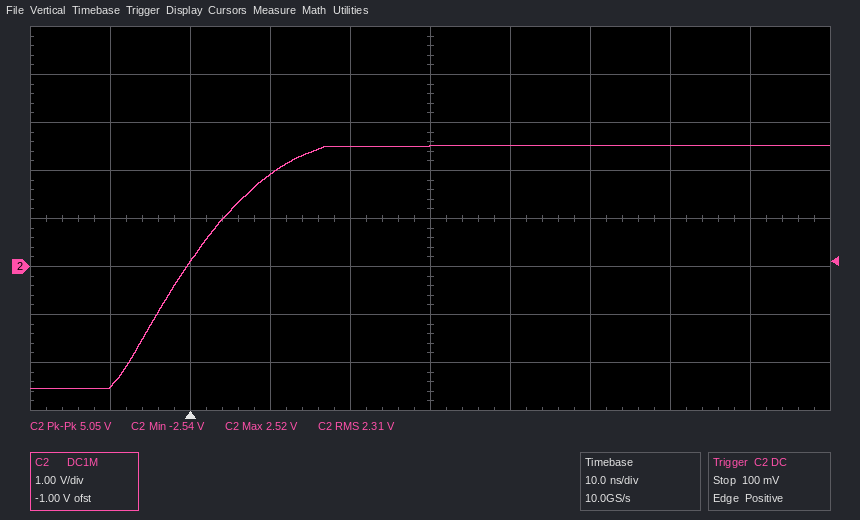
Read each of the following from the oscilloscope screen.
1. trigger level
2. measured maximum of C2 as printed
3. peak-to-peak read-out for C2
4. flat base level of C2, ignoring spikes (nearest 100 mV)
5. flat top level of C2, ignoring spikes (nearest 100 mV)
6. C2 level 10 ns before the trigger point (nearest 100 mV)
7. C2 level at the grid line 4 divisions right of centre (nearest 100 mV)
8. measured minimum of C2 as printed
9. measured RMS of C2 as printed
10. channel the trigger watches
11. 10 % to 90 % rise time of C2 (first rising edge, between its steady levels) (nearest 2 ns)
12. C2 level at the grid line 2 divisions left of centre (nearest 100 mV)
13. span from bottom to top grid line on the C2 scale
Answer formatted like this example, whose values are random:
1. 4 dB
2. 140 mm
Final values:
1. 100 mV
2. 2.52 V
3. 5.05 V
4. -2.5 V
5. 2.5 V
6. -2.5 V
7. 2.5 V
8. -2.54 V
9. 2.31 V
10. C2
11. 18 ns
12. 1.9 V
13. 8 V
